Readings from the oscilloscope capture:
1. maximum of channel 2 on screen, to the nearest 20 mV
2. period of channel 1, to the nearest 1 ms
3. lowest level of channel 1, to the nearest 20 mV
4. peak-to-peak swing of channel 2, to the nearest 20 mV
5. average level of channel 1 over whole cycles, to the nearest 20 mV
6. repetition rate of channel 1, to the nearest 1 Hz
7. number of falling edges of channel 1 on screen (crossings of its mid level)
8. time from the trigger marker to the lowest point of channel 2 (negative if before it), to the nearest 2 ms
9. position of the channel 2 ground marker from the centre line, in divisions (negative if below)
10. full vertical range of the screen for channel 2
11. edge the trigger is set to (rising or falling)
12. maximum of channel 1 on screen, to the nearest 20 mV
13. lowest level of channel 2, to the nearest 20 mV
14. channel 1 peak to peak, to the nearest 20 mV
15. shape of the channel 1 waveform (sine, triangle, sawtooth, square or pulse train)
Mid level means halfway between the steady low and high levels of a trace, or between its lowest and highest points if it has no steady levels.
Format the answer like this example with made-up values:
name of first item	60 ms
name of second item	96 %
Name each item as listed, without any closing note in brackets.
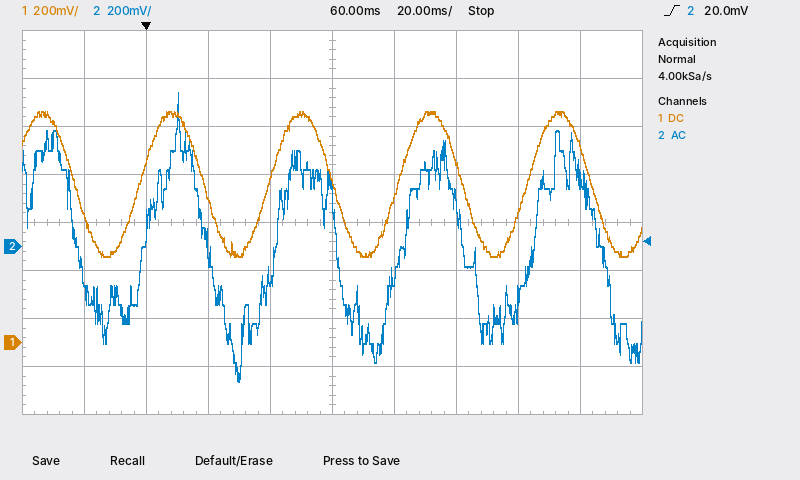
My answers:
maximum of channel 2 on screen, to the nearest 20 mV	640 mV
period of channel 1, to the nearest 1 ms	42 ms
lowest level of channel 1, to the nearest 20 mV	360 mV
peak-to-peak swing of channel 2, to the nearest 20 mV	1.20 V
average level of channel 1 over whole cycles, to the nearest 20 mV	660 mV
repetition rate of channel 1, to the nearest 1 Hz	24 Hz
number of falling edges of channel 1 on screen	5
time from the trigger marker to the lowest point of channel 2 (negative if before it), to the nearest 2 ms	+30 ms
position of the channel 2 ground marker from the centre line, in divisions	-0.5 div
full vertical range of the screen for channel 2	1.6 V
edge the trigger is set to	rising
maximum of channel 1 on screen, to the nearest 20 mV	960 mV
lowest level of channel 2, to the nearest 20 mV	-560 mV
channel 1 peak to peak, to the nearest 20 mV	600 mV
shape of the channel 1 waveform	sine
